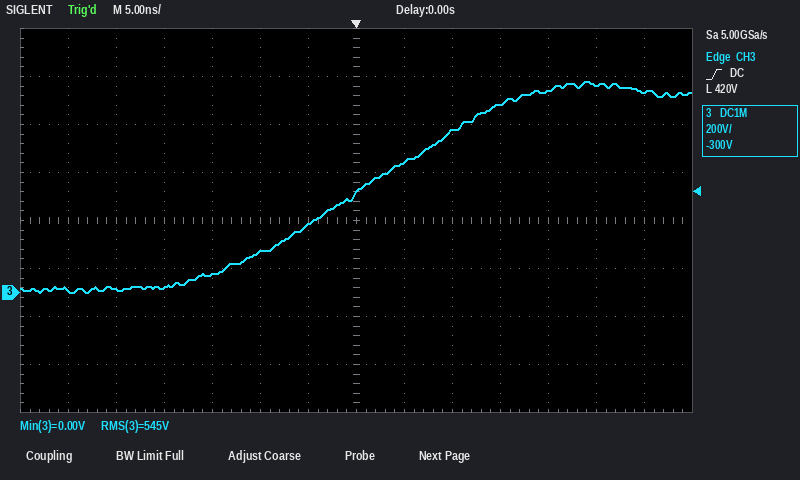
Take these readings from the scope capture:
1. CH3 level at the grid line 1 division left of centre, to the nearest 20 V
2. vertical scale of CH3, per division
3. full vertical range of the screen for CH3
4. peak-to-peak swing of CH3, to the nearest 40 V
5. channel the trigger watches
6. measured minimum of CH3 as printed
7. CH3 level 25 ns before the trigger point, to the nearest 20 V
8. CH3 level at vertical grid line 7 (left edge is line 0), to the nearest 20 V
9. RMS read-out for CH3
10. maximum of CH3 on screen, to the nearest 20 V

280 V
200 V
1.6 kV
880 V
CH3
0.00 V
20 V
420 V
545 V
880 V
